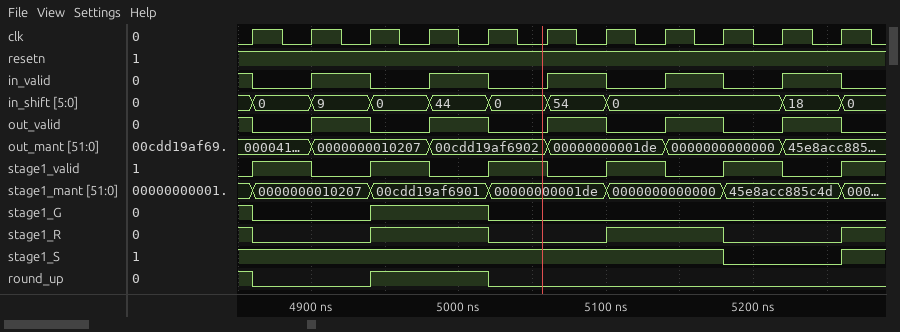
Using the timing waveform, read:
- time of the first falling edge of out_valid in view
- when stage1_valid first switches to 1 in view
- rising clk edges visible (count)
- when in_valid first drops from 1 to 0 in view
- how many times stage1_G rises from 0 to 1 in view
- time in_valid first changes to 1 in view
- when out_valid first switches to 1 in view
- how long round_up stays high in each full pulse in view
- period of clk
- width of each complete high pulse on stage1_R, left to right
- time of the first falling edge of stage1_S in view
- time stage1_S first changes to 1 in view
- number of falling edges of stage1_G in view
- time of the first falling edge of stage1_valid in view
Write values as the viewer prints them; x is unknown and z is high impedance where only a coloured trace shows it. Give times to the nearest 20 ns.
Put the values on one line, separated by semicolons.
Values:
4860 ns; 4860 ns; 11; 4860 ns; 1; 4900 ns; 4900 ns; 80 ns; 40 ns; 80 ns, 80 ns; 5180 ns; 5260 ns; 2; 4900 ns
